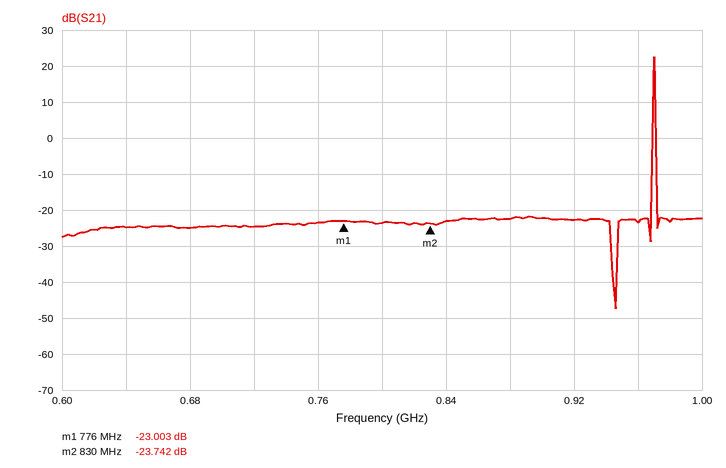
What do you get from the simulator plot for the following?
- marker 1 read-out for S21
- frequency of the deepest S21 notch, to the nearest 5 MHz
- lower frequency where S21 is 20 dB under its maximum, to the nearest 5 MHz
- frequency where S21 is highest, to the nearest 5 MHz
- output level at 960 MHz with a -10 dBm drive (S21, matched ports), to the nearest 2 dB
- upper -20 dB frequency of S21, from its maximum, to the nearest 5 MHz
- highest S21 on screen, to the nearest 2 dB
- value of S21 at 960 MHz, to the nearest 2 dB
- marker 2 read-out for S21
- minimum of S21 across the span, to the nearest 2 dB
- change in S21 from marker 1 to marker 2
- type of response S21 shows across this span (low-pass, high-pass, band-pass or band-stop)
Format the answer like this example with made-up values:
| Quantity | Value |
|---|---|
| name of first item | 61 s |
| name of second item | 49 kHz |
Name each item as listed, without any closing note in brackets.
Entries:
| Quantity | Value |
|---|---|
| marker 1 read-out for S21 | -23.003 dB |
| frequency of the deepest S21 notch, to the nearest 5 MHz | 945 MHz |
| lower frequency where S21 is 20 dB under its maximum, to the nearest 5 MHz | 970 MHz |
| frequency where S21 is highest, to the nearest 5 MHz | 970 MHz |
| output level at 960 MHz with a -10 dBm drive (S21, matched ports), to the nearest 2 dB | -34 dBm |
| upper -20 dB frequency of S21, from its maximum, to the nearest 5 MHz | 970 MHz |
| highest S21 on screen, to the nearest 2 dB | 22 dB |
| value of S21 at 960 MHz, to the nearest 2 dB | -24 dB |
| marker 2 read-out for S21 | -23.742 dB |
| minimum of S21 across the span, to the nearest 2 dB | -48 dB |
| change in S21 from marker 1 to marker 2 | -0.739 dB |
| type of response S21 shows across this span | band-pass |
